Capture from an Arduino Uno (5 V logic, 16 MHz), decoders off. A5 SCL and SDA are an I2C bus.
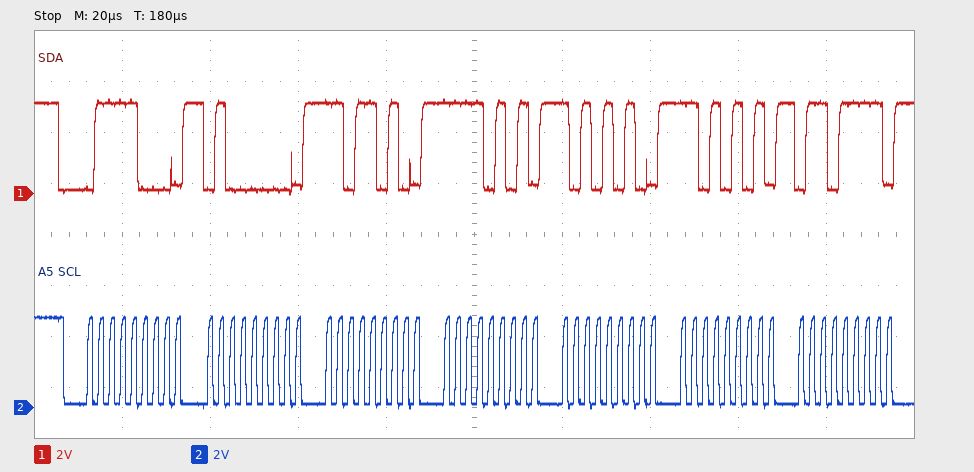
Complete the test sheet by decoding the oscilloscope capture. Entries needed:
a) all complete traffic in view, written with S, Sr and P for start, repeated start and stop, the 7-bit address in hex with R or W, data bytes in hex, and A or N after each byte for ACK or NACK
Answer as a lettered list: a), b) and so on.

a) S 3CW A 40 A DA A F5 A AA A D5 A 6F A
